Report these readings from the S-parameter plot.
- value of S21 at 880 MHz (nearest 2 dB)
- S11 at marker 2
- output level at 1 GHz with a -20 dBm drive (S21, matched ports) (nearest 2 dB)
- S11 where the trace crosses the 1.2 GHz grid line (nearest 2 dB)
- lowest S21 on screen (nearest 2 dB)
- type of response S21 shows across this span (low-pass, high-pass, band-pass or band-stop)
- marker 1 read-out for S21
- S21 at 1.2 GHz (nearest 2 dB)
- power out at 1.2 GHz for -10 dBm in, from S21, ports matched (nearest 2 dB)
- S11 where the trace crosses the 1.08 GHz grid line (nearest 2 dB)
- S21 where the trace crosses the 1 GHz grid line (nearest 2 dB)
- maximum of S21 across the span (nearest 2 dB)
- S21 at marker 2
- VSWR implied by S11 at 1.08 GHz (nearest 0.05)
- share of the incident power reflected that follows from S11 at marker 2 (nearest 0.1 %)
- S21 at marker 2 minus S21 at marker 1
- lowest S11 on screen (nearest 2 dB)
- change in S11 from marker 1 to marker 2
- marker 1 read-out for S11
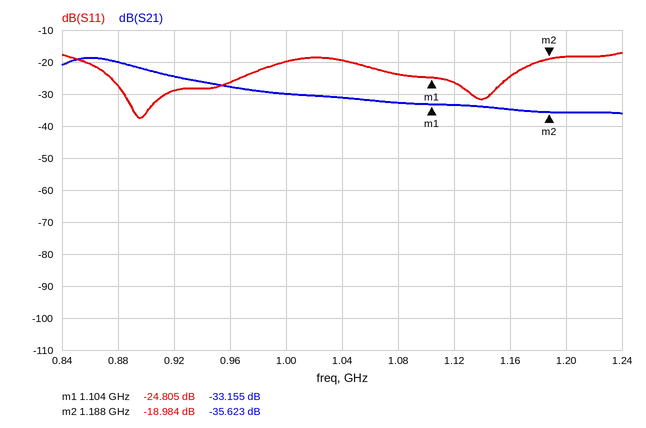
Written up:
-20 dB
-18.984 dB
-50 dBm
-18 dB
-36 dB
low-pass
-33.155 dB
-36 dB
-46 dBm
-24 dB
-30 dB
-18 dB
-35.623 dB
1.15
1.3 %
-2.468 dB
-38 dB
5.821 dB
-24.805 dB
